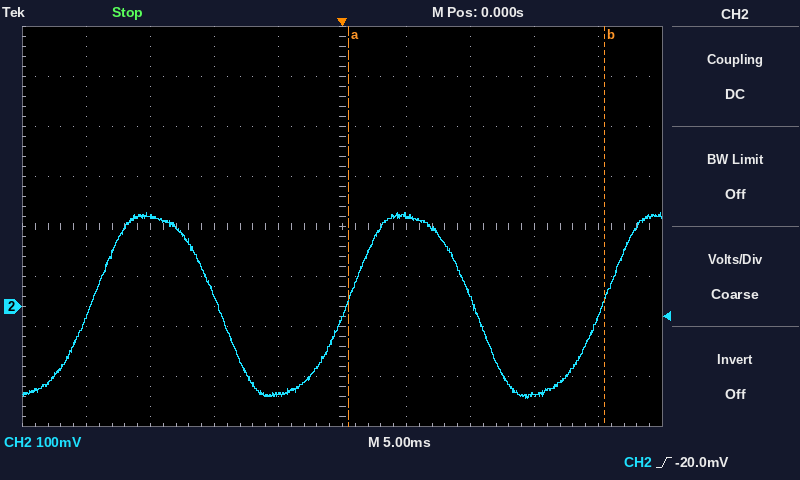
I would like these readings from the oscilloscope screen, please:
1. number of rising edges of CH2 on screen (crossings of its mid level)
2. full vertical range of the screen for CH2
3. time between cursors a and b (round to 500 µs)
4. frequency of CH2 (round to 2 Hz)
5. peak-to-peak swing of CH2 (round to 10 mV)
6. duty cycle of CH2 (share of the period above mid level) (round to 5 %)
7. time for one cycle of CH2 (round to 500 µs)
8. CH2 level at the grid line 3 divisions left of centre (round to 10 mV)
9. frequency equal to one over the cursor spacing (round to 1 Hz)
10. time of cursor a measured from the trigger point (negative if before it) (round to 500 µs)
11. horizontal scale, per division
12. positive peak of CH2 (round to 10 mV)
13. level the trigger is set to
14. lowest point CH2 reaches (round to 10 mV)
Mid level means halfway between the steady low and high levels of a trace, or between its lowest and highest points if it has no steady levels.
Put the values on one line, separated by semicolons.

3; 800 mV; 20.0 ms; 50 Hz; 370 mV; 50 %; 20.0 ms; 180 mV; 50 Hz; +500 µs; 5 ms; 190 mV; -20.0 mV; -180 mV
